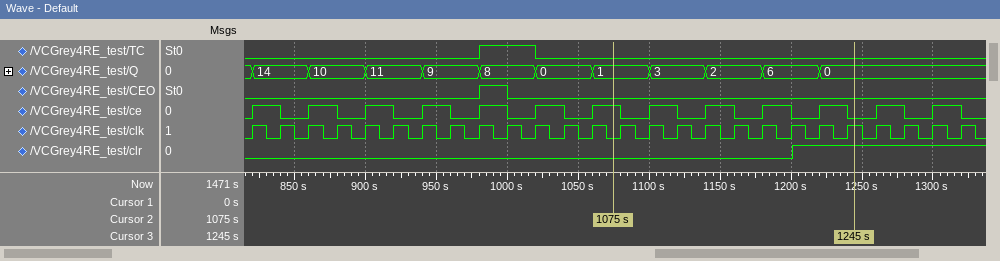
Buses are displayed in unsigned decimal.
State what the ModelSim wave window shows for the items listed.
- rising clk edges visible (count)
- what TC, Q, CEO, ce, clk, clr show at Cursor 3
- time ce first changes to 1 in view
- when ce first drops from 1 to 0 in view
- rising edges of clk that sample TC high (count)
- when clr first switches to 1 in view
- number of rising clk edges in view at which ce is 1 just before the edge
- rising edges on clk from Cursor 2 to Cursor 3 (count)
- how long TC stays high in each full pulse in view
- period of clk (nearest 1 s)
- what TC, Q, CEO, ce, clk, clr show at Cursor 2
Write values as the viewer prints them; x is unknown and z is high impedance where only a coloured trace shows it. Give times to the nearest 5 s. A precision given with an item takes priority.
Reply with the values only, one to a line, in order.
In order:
26
TC=0, Q=0, CEO=0, ce=0, clk=1, clr=1
820 s
840 s
2
1200 s
13
9
40 s
20 s
TC=0, Q=1, CEO=0, ce=1, clk=0, clr=0
